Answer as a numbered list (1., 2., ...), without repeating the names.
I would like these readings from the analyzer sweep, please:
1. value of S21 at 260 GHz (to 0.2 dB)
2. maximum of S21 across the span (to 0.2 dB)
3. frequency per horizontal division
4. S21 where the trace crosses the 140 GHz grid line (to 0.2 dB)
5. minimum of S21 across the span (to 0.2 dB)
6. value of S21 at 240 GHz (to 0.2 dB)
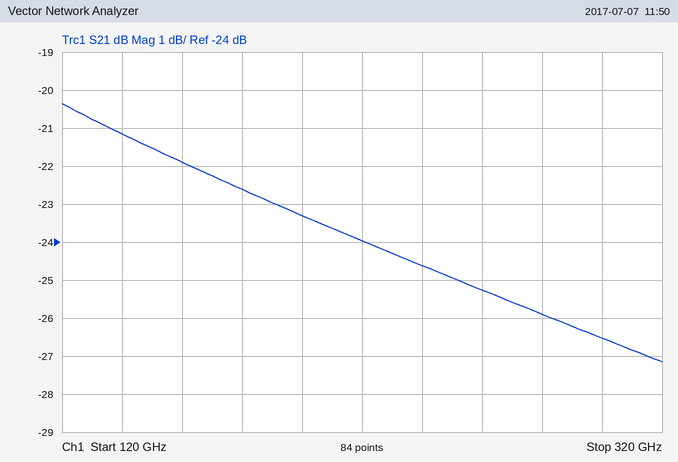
1. -25.2 dB
2. -20.4 dB
3. 20 GHz
4. -21.2 dB
5. -27.2 dB
6. -24.6 dB
